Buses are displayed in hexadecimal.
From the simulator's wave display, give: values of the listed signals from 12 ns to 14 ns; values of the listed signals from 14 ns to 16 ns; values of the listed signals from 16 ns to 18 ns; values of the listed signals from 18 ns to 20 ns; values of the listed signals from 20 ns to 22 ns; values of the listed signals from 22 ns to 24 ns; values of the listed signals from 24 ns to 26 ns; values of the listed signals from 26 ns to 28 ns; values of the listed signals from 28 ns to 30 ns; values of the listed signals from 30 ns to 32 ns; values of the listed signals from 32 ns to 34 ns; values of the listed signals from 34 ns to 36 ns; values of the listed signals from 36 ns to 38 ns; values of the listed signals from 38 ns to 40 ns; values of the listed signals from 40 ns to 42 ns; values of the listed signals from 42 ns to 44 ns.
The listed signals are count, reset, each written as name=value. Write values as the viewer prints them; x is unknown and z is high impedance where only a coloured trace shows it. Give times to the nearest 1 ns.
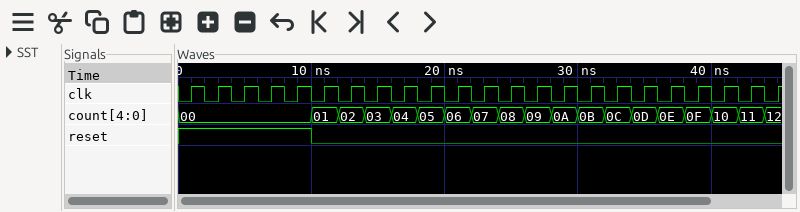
count=02, reset=0
count=03, reset=0
count=04, reset=0
count=05, reset=0
count=06, reset=0
count=07, reset=0
count=08, reset=0
count=09, reset=0
count=0A, reset=0
count=0B, reset=0
count=0C, reset=0
count=0D, reset=0
count=0E, reset=0
count=0F, reset=0
count=10, reset=0
count=11, reset=0
